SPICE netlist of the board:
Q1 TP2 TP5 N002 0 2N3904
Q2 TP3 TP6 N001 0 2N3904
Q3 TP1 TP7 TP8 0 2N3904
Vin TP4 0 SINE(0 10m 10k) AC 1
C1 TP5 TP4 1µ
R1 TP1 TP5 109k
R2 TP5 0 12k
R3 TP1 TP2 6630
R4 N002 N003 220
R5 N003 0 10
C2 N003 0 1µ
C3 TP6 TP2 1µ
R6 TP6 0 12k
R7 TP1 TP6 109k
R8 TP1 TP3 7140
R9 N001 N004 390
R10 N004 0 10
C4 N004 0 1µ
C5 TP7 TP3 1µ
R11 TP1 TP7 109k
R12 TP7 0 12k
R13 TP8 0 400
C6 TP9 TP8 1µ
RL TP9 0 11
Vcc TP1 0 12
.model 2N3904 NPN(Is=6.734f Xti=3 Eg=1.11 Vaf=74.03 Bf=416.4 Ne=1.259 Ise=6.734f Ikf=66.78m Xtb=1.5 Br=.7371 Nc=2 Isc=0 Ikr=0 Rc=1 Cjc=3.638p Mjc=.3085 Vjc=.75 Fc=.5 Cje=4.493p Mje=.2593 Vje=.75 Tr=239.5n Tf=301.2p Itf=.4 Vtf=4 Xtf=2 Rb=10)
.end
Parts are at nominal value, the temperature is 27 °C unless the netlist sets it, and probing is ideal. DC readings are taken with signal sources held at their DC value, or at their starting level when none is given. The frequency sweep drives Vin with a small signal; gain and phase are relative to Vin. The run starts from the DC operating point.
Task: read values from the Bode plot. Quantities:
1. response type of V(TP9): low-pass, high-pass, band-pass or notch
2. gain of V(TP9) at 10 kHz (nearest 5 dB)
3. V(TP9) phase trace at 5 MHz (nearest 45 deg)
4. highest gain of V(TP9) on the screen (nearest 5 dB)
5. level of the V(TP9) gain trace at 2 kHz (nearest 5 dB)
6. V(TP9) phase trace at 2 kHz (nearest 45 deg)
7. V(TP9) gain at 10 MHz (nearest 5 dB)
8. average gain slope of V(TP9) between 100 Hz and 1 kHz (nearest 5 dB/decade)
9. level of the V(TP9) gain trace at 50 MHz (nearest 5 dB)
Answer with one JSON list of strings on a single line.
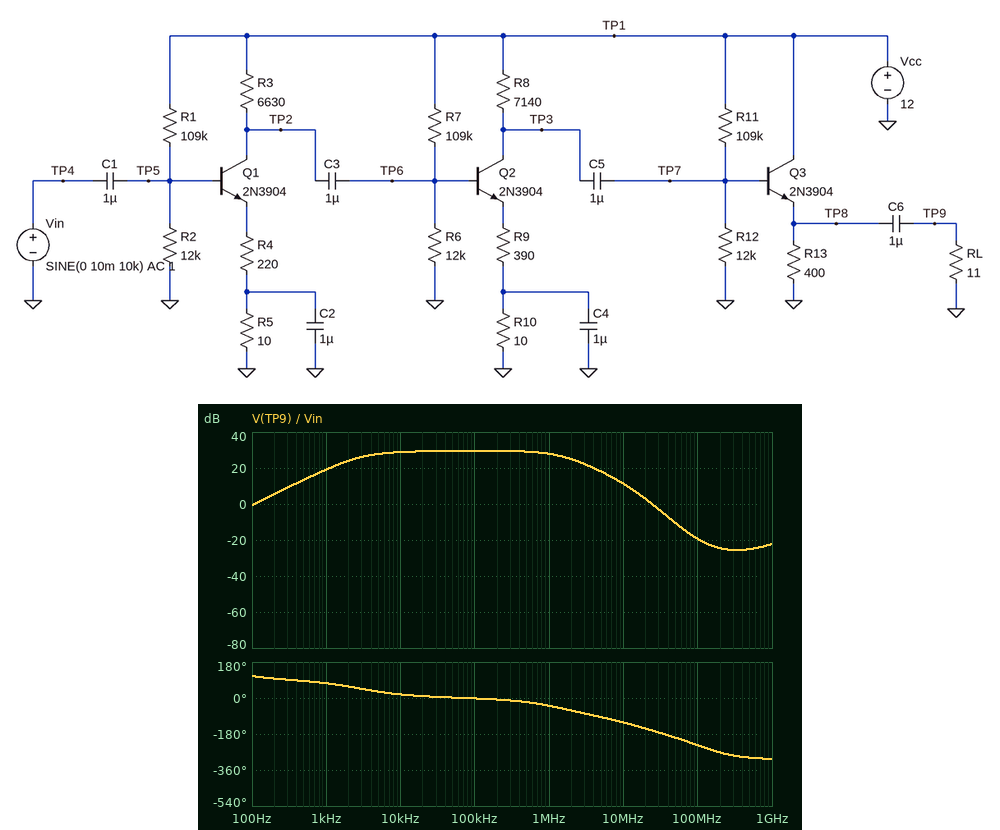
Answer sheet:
["band-pass", "30 dB", "-90 deg", "30 dB", "25 dB", "45 deg", "10 dB", "20 dB/decade", "-10 dB"]
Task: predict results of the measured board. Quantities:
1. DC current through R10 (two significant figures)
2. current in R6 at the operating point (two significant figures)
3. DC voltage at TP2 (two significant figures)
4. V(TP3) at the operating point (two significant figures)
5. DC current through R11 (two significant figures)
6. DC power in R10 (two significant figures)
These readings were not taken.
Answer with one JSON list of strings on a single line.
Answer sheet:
["1.1 mA", "92 µA", "1.0 V", "4.2 V", "100 µA", "12 µW"]
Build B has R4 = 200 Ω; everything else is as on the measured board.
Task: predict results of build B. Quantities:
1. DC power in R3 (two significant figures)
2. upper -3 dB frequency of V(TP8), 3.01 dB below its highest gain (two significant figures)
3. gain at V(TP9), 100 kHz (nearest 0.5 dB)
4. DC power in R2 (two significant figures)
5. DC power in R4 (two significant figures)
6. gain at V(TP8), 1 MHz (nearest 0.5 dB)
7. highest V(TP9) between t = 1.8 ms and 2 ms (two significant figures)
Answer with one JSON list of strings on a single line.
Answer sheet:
["20 mW", "3.4 kHz", "29.0 dB", "91 µW", "600 µW", "27.0 dB", "82 mV"]
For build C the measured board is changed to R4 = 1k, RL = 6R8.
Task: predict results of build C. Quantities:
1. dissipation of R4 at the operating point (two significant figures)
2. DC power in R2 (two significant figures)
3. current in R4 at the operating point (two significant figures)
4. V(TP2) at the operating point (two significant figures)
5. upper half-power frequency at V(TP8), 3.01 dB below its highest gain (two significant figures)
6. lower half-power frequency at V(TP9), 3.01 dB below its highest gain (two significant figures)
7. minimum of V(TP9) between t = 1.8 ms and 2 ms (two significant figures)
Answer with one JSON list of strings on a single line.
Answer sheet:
["250 µW", "110 µW", "500 µA", "8.7 V", "3.3 kHz", "3.4 kHz", "-11 mV"]
